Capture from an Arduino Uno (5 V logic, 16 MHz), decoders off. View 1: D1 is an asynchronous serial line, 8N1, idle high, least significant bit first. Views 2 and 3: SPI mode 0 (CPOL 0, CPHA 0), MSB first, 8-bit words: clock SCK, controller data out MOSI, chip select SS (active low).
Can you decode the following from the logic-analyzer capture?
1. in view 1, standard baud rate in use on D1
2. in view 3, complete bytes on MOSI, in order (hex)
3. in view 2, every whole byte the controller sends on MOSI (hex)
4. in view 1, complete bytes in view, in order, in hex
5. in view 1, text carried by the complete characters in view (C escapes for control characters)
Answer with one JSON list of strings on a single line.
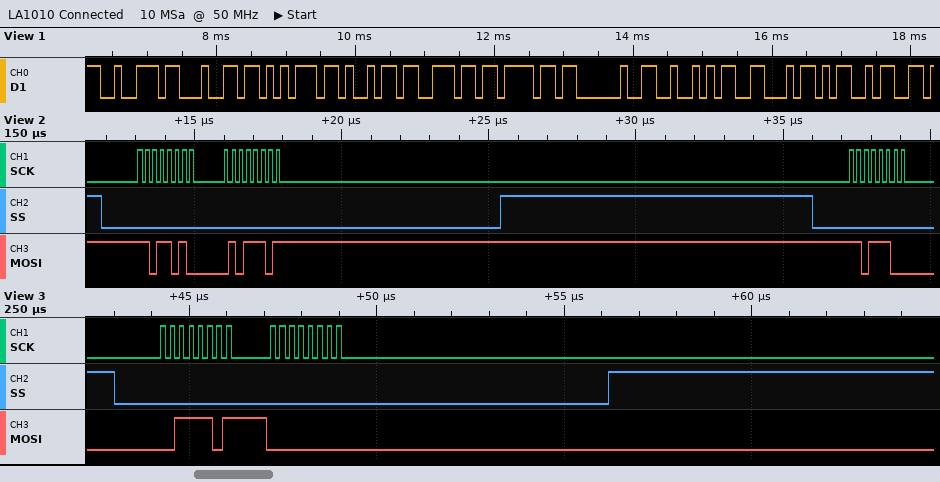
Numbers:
["9600 baud", "0x3D 0x00", "DA 5D DC", "72 64 75 69 6E 6F 20 52 46 4D", "\"rduino RFM\""]
